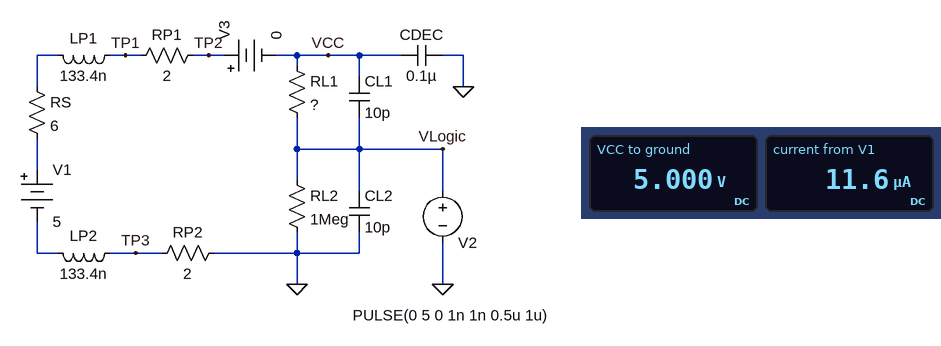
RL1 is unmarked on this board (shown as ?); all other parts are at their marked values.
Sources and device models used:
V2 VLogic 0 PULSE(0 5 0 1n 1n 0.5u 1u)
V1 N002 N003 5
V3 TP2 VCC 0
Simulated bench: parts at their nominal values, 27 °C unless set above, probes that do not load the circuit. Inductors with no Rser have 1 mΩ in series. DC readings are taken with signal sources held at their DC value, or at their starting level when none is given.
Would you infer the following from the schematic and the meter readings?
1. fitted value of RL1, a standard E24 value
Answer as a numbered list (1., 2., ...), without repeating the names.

1. 430 kΩ
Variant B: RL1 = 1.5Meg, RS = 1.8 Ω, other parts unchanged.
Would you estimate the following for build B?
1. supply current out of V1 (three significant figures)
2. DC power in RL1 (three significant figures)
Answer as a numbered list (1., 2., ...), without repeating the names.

1. 3.33 µA
2. 16.7 µW
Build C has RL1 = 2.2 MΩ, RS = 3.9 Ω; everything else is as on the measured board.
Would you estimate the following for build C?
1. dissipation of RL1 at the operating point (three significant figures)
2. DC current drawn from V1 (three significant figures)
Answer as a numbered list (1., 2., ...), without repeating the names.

1. 11.4 µW
2. 2.27 µA
